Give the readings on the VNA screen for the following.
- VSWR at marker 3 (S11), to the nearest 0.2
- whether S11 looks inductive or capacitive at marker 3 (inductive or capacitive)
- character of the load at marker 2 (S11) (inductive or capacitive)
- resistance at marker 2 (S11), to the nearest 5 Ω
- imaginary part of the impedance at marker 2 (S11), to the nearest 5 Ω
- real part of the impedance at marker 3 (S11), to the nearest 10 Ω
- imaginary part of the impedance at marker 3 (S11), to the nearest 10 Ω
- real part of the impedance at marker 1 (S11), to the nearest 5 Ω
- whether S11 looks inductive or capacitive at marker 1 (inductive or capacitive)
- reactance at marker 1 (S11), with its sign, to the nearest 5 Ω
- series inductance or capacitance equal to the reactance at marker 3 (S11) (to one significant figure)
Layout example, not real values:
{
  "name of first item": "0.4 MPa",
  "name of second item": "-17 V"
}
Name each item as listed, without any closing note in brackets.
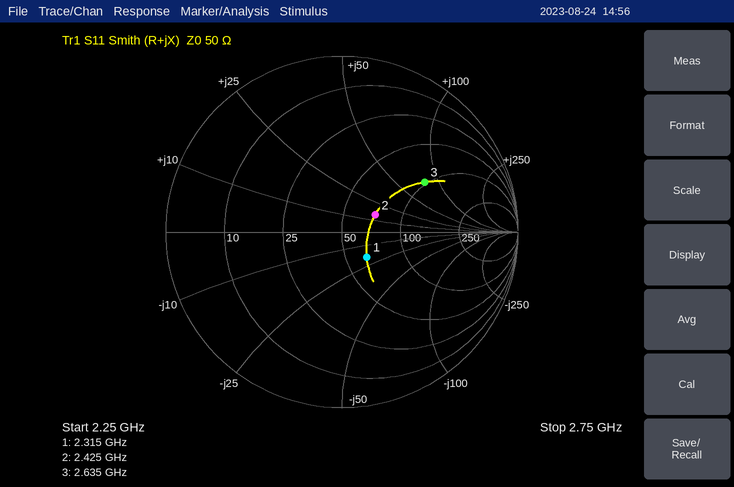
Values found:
{
  "VSWR at marker 3 (S11), to the nearest 0.2": "3.4",
  "whether S11 looks inductive or capacitive at marker 3": "inductive",
  "character of the load at marker 2 (S11)": "inductive",
  "resistance at marker 2 (S11), to the nearest 5 Ω": "70 Ω",
  "imaginary part of the impedance at marker 2 (S11), to the nearest 5 Ω": "+15 Ω",
  "real part of the impedance at marker 3 (S11), to the nearest 10 Ω": "100 Ω",
  "imaginary part of the impedance at marker 3 (S11), to the nearest 10 Ω": "+80 Ω",
  "real part of the impedance at marker 1 (S11), to the nearest 5 Ω": "65 Ω",
  "whether S11 looks inductive or capacitive at marker 1": "capacitive",
  "reactance at marker 1 (S11), with its sign, to the nearest 5 Ω": "-20 Ω",
  "series inductance or capacitance equal to the reactance at marker 3 (S11)": "5 nH"
}
